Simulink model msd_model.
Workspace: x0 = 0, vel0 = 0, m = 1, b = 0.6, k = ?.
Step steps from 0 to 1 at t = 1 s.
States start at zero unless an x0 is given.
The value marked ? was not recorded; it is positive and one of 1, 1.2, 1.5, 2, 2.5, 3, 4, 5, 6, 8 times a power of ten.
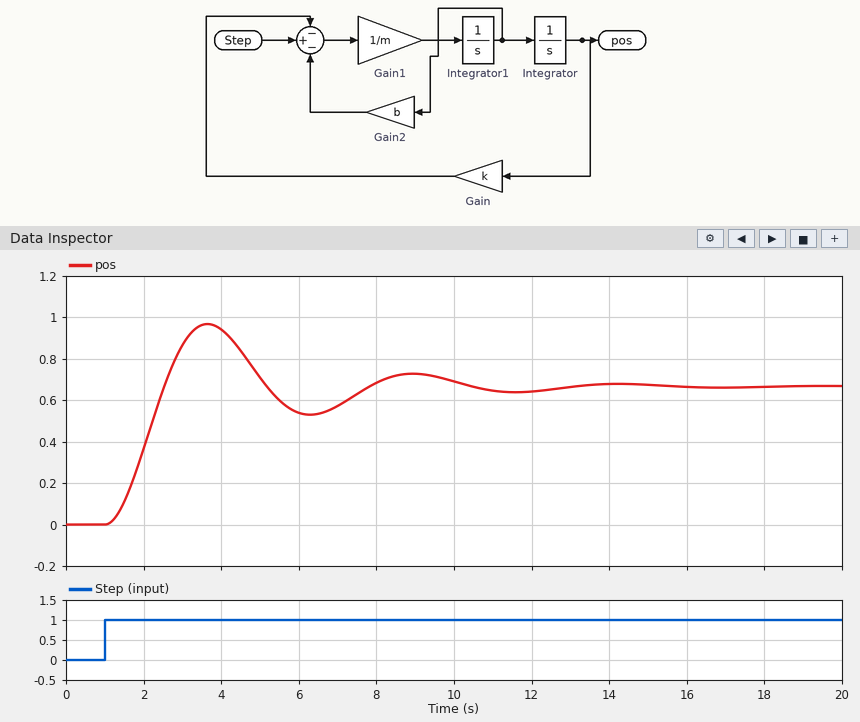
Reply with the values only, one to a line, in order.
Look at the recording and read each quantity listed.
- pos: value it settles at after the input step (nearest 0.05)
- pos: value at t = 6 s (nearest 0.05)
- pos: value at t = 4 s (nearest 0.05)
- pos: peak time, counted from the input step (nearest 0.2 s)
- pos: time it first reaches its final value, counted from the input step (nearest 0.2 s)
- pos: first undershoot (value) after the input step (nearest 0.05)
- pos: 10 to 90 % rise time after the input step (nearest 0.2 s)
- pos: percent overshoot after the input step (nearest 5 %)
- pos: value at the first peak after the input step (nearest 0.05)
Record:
0.65
0.55
0.95
2.6 s
1.6 s
0.55
1.0 s
45 %
0.95
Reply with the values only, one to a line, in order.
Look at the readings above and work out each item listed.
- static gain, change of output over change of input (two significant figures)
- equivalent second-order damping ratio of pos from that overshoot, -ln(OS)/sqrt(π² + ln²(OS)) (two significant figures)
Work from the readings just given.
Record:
0.65
0.25
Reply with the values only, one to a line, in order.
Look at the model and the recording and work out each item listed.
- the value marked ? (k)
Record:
1.5
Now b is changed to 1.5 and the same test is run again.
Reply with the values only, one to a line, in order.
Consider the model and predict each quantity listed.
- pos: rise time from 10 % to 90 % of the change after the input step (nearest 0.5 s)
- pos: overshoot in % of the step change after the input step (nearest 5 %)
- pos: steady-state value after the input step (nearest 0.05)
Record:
1.5 s
10 %
0.65
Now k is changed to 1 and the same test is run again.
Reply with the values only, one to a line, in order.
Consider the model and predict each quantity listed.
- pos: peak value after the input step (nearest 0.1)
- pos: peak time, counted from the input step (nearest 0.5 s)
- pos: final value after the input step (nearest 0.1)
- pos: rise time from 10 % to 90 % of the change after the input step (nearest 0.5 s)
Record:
1.4
3.5 s
1.0
1.5 s
